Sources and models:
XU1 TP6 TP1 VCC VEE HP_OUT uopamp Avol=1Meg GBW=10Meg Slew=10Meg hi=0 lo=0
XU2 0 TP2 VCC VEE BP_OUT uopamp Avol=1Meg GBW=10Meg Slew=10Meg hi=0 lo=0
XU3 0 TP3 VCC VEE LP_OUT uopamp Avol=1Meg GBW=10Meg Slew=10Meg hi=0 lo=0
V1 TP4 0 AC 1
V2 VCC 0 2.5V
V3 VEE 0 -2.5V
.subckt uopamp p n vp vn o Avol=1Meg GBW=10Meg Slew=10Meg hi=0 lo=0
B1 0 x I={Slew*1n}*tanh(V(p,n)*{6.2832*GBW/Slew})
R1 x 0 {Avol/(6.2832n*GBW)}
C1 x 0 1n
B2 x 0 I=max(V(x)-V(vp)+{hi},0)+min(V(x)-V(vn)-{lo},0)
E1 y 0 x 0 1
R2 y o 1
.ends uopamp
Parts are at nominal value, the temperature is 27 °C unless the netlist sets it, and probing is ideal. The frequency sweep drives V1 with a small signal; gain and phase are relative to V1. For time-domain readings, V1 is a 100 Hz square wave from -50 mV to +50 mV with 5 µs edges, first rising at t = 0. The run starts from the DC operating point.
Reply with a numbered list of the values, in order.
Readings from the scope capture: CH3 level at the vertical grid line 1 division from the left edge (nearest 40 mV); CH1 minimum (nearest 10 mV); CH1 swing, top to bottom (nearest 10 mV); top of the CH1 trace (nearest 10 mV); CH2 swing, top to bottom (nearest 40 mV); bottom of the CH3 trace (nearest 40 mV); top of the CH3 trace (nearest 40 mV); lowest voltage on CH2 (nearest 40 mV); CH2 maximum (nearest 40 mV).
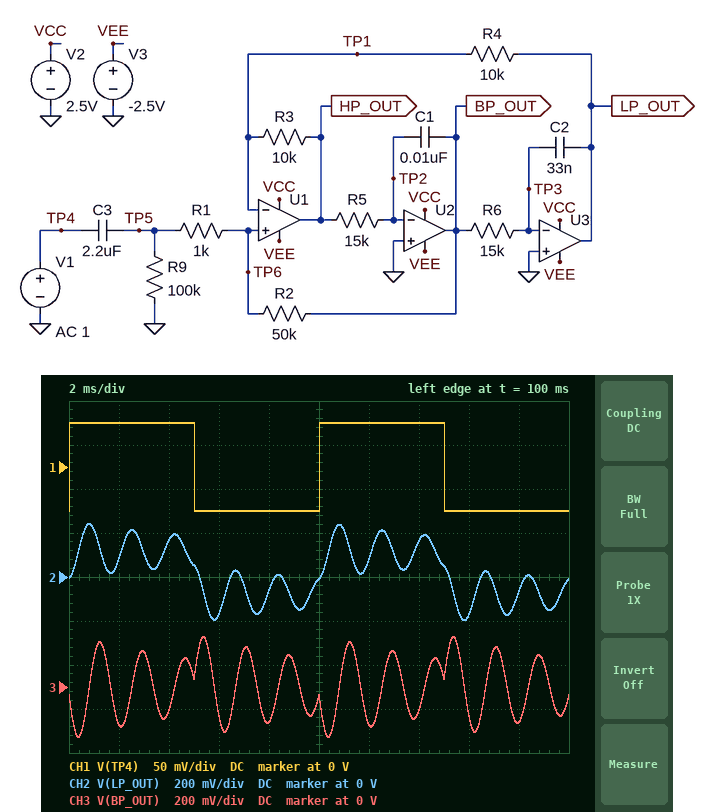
1. -160 mV
2. -50 mV
3. 100 mV
4. 50 mV
5. 440 mV
6. -240 mV
7. 240 mV
8. -200 mV
9. 240 mV
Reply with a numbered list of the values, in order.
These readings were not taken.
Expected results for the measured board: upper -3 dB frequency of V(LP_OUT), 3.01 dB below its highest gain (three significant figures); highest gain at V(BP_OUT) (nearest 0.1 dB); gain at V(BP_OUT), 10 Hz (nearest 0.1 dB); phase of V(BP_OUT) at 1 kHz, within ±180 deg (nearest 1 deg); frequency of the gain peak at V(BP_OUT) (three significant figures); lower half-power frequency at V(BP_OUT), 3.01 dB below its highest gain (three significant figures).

1. 606 Hz
2. 34.0 dB
3. -24.6 dB
4. 94 deg
5. 587 Hz
6. 566 Hz
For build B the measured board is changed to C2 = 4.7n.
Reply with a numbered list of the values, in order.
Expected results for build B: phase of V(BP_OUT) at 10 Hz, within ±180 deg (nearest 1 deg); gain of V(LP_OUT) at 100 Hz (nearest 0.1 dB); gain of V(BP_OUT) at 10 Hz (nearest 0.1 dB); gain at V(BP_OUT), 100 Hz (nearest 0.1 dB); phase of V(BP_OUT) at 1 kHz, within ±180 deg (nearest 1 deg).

1. -78 deg
2. 5.9 dB
3. -41.4 dB
4. -21.2 dB
5. -92 deg
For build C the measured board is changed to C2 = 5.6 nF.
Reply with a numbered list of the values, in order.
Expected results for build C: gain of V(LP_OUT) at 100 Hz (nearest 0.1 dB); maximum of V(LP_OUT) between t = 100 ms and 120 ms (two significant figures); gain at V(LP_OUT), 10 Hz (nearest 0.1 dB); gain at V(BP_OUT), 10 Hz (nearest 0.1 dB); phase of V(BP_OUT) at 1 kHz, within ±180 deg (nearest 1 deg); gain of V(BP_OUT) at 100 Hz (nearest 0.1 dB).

1. 5.9 dB
2. 250 mV
3. 5.6 dB
4. -39.9 dB
5. -92 deg
6. -19.7 dB
